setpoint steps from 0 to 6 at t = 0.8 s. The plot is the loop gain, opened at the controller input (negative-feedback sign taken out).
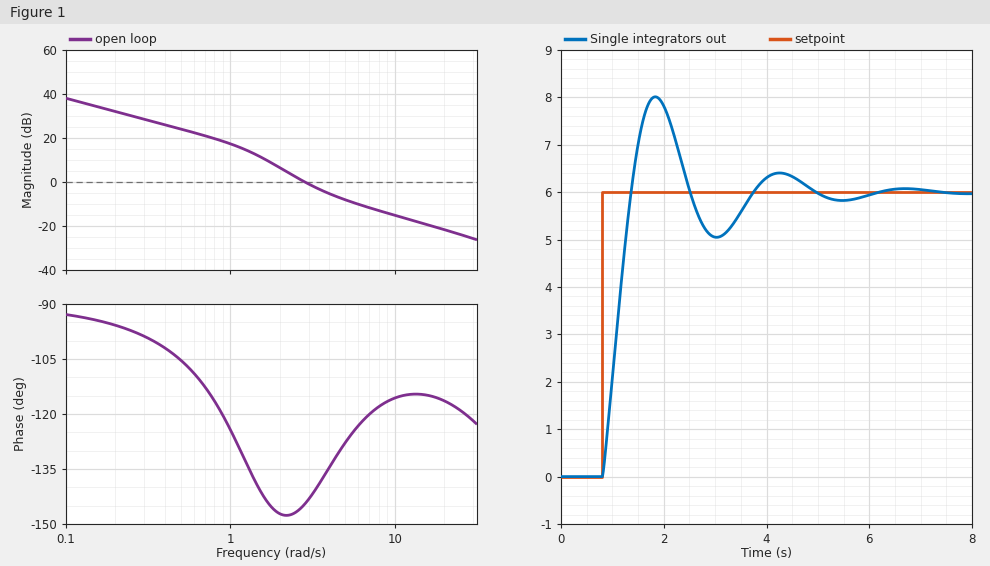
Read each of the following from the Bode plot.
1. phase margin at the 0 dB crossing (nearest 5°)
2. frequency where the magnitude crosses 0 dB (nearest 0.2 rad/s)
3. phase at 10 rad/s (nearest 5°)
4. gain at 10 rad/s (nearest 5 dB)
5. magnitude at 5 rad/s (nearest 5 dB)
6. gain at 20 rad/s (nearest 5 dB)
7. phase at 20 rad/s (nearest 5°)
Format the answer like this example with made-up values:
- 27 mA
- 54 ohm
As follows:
- 35°
- 2.8 rad/s
- -115°
- -15 dB
- -10 dB
- -20 dB
- -115°
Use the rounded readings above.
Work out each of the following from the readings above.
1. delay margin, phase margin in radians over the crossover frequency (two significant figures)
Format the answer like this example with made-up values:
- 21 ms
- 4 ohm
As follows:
- 0.22 s
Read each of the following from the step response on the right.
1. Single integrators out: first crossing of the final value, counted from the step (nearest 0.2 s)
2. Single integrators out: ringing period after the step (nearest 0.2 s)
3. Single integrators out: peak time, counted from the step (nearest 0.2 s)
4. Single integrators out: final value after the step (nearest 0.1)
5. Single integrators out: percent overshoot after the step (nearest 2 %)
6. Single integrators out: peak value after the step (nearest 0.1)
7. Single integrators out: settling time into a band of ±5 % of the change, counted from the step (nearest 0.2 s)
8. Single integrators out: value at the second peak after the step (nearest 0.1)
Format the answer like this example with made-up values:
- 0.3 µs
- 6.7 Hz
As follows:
- 0.6 s
- 2.4 s
- 1.0 s
- 6.0
- 34 %
- 8.0
- 3.8 s
- 6.4
